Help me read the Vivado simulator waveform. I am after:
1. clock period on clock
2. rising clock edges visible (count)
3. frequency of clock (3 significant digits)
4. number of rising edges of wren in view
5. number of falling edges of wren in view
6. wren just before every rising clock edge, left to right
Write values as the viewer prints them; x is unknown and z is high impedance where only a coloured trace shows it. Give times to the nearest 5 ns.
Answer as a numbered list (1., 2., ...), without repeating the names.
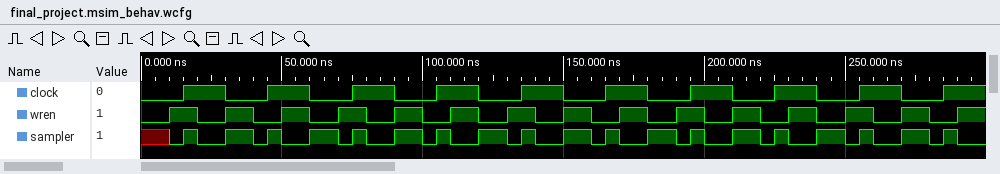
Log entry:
1. 30 ns
2. 10
3. 33.3 MHz
4. 15
5. 14
6. 1 0 1 0 1 0 1 0 1 0
